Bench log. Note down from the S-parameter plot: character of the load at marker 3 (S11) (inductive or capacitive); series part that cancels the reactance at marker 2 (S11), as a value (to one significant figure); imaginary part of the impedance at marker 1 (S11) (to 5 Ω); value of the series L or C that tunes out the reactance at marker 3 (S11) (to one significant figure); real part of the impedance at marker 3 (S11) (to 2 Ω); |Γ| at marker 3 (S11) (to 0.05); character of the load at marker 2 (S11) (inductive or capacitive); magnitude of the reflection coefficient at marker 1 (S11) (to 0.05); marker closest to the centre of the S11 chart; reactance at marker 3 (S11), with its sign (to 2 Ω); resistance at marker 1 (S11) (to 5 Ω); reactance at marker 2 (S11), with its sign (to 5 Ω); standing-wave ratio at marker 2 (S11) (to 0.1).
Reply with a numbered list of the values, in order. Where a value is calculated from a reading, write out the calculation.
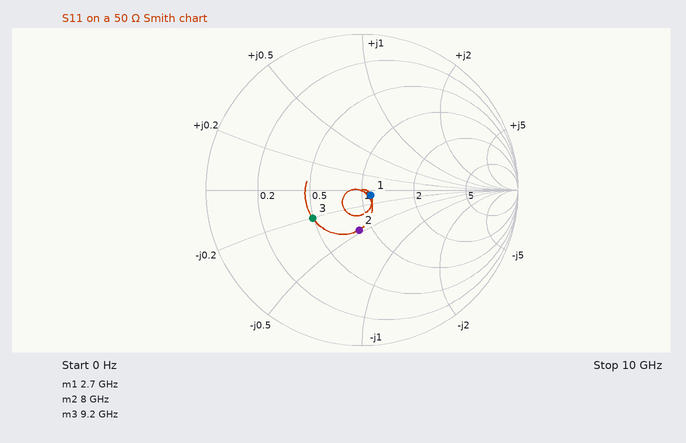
1. capacitive
2. L = 25 Ω/(2π × 8 GHz) ≈ 497 pH, so 500 pH to one significant figure
3. -5 Ω
4. L = 10 Ω/(2π × 9.2 GHz) ≈ 173 pH, so 200 pH to one significant figure
5. 24 Ω
6. 0.35
7. capacitive
8. 0.05
9. marker 1
10. -10 Ω
11. 55 Ω
12. -25 Ω
13. 1.7
